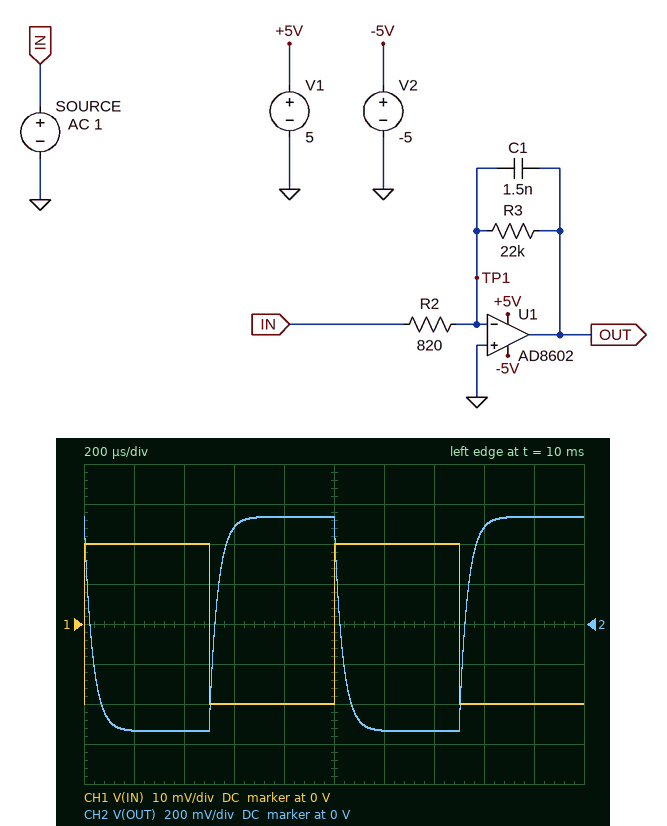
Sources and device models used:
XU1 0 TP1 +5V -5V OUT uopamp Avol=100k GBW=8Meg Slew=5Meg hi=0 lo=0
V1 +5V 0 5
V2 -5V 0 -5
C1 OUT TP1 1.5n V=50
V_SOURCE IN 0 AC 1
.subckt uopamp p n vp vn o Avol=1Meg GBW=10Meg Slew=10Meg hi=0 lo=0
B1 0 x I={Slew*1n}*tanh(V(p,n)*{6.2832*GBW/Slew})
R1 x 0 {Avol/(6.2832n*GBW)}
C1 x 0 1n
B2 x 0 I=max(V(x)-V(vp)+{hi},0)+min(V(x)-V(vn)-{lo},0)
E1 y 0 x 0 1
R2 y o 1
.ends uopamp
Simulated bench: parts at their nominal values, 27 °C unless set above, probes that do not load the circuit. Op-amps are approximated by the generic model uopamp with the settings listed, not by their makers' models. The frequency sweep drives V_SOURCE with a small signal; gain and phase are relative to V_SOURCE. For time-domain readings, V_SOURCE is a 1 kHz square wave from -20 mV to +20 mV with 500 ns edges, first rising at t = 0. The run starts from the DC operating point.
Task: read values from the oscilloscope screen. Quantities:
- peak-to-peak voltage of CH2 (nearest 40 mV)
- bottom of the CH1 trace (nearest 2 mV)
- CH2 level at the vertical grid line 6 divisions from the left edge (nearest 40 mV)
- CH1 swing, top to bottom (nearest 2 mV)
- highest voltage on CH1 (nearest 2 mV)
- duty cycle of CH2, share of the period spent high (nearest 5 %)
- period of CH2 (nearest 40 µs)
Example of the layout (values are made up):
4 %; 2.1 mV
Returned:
1.08 V; -20 mV; -520 mV; 40 mV; 20 mV; 50 %; 1.00 ms
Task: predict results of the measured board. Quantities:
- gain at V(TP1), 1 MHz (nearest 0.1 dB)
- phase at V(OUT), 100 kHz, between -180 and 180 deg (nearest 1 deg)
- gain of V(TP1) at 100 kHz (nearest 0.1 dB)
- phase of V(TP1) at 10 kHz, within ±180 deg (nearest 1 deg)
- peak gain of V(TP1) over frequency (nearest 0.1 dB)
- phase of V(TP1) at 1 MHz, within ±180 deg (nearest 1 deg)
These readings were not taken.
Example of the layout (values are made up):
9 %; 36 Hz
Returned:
-36.0 dB; 92 deg; -36.0 dB; 25 deg; -36.0 dB; -6 deg
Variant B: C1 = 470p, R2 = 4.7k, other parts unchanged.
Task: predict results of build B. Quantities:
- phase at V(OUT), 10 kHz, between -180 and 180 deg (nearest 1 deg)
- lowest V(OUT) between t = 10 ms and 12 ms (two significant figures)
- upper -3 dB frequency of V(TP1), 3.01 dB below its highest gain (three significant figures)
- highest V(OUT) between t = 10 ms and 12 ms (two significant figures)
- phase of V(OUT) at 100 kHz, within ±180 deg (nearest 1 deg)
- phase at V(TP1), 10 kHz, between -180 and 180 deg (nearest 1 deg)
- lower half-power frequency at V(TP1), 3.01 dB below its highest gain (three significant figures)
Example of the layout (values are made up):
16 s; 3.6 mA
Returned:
147 deg; -94 mV; 8.11 MHz; 94 mV; 98 deg; 56 deg; 15.2 kHz
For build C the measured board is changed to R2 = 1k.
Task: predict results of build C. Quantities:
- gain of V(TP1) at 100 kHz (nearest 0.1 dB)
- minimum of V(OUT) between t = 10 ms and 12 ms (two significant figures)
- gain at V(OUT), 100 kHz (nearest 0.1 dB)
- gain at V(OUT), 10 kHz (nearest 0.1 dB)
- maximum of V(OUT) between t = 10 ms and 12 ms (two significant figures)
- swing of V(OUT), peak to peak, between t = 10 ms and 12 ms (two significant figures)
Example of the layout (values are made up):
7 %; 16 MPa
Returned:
-37.7 dB; -440 mV; 0.4 dB; 19.5 dB; 440 mV; 880 mV
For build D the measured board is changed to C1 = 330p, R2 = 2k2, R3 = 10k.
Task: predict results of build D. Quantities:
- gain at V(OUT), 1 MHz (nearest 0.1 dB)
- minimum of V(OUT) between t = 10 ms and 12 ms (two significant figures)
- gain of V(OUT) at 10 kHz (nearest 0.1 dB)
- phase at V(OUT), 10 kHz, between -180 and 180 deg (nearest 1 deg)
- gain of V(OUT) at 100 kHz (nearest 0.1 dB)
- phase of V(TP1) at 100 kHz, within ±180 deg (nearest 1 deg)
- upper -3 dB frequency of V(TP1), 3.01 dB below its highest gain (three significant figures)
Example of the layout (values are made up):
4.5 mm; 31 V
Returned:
-13.5 dB; -91 mV; 13.0 dB; 168 deg; 5.7 dB; 24 deg; 8.31 MHz
